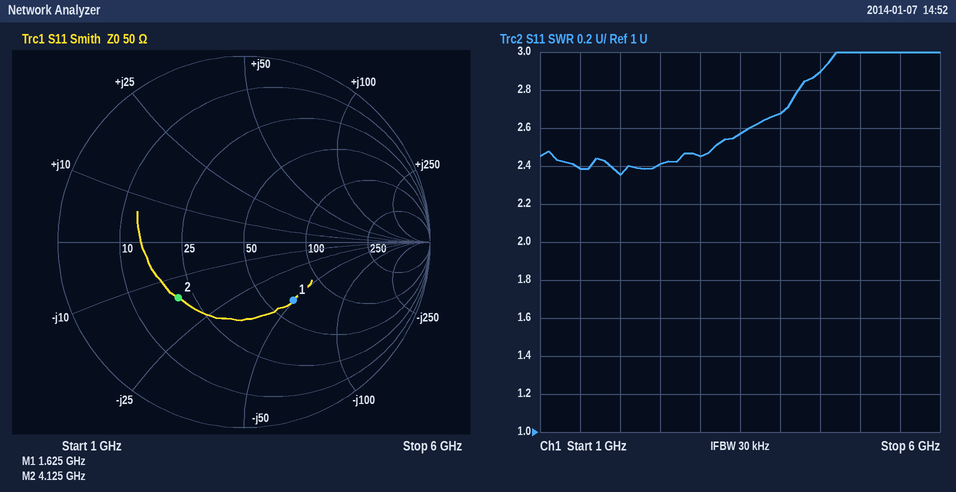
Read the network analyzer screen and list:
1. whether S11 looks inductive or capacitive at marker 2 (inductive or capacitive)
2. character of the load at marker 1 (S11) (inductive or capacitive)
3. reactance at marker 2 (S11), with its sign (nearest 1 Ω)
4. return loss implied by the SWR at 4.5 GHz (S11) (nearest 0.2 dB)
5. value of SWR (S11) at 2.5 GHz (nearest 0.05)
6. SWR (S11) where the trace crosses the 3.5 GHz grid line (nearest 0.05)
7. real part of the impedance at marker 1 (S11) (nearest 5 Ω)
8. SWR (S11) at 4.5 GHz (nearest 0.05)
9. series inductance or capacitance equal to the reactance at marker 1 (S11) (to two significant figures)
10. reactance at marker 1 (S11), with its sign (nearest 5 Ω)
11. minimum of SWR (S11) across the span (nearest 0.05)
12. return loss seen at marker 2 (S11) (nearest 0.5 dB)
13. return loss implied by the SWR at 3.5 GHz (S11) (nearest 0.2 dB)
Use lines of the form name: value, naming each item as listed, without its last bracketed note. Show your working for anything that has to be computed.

whether S11 looks inductive or capacitive at marker 2: capacitive
character of the load at marker 1 (S11): capacitive
reactance at marker 2 (S11), with its sign: -16 Ω
return loss implied by the SWR at 4.5 GHz (S11): −20 log10((2.9 − 1)/(2.9 + 1)) ≈ 6.2 dB
value of SWR (S11) at 2.5 GHz: 2.40
SWR (S11) where the trace crosses the 3.5 GHz grid line: 2.55
real part of the impedance at marker 1 (S11): 65 Ω
SWR (S11) at 4.5 GHz: 2.90
series inductance or capacitance equal to the reactance at marker 1 (S11): C = 1/(2π × 1.625 GHz × 50 Ω) ≈ 2.0 pF
reactance at marker 1 (S11), with its sign: -50 Ω
minimum of SWR (S11) across the span: 2.35
return loss seen at marker 2 (S11): 6.5 dB
return loss implied by the SWR at 3.5 GHz (S11): −20 log10((2.55 − 1)/(2.55 + 1)) ≈ 7.2 dB
